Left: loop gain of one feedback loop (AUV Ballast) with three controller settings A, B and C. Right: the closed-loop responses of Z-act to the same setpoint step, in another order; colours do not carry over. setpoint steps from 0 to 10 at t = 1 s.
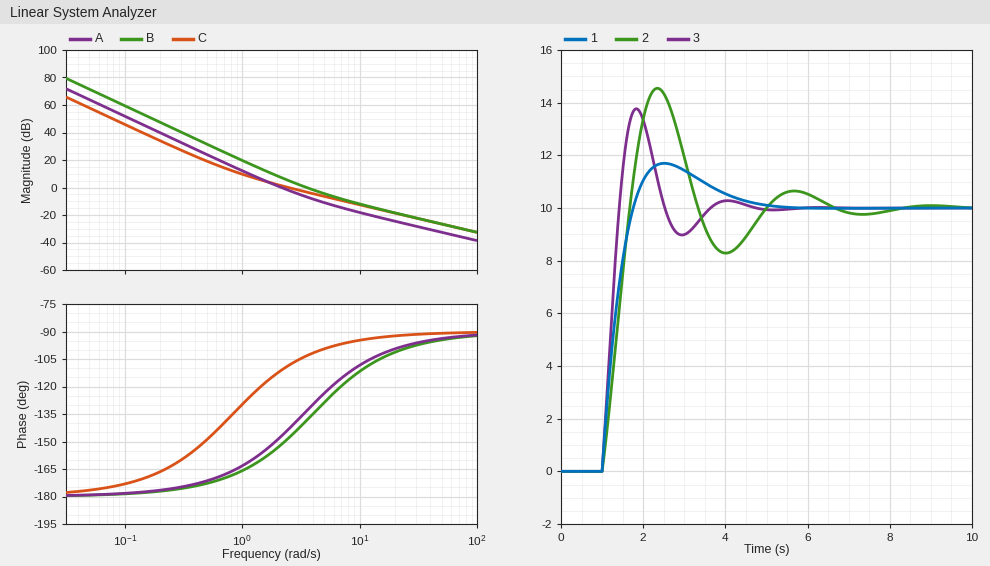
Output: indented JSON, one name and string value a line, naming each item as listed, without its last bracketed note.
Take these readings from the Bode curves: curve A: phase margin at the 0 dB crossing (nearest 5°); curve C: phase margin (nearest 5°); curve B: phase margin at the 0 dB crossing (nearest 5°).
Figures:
{
  "curve A: phase margin at the 0 dB crossing": "35°",
  "curve C: phase margin": "70°",
  "curve B: phase margin at the 0 dB crossing": "40°"
}
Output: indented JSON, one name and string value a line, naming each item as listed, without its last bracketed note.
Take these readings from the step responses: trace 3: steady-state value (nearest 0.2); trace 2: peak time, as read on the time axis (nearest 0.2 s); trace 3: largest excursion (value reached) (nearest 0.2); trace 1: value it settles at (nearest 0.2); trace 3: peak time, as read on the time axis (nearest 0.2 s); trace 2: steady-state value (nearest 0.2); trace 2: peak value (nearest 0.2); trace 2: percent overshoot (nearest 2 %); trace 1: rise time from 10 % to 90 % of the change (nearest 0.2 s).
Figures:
{
  "trace 3: steady-state value": "10.0",
  "trace 2: peak time, as read on the time axis": "2.4 s",
  "trace 3: largest excursion (value reached)": "13.8",
  "trace 1: value it settles at": "10.0",
  "trace 3: peak time, as read on the time axis": "1.8 s",
  "trace 2: steady-state value": "10.0",
  "trace 2: peak value": "14.6",
  "trace 2: percent overshoot": "46 %",
  "trace 1: rise time from 10 % to 90 % of the change": "0.6 s"
}
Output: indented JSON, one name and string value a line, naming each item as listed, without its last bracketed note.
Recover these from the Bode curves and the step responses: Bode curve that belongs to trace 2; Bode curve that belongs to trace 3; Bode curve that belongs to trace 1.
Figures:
{
  "Bode curve that belongs to trace 2": "A",
  "Bode curve that belongs to trace 3": "B",
  "Bode curve that belongs to trace 1": "C"
}
